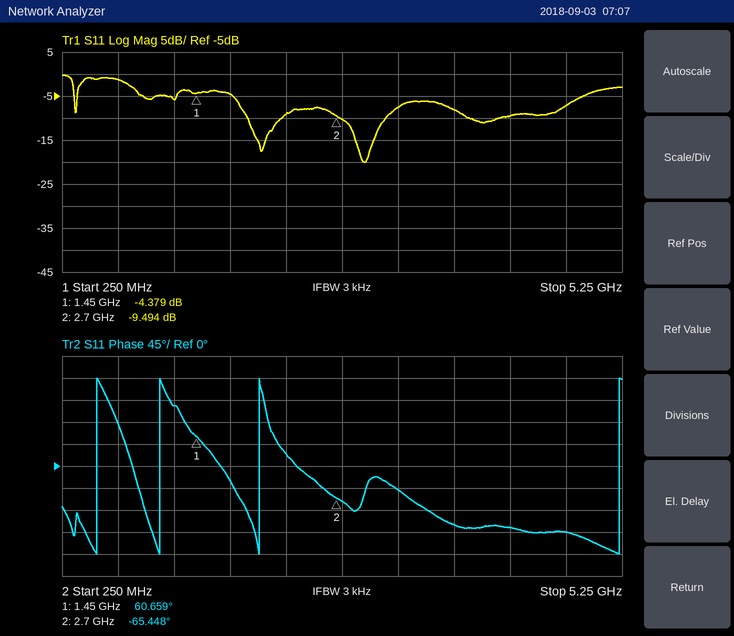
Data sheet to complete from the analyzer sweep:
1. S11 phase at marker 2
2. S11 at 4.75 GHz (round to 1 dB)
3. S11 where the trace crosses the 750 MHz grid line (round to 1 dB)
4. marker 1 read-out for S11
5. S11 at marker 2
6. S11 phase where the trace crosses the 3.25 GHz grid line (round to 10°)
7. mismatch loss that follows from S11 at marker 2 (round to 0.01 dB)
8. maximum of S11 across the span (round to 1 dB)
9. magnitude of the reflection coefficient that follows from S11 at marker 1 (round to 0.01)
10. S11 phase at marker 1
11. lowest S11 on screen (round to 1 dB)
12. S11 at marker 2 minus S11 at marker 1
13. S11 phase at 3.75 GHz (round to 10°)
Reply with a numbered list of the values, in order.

1. -65.448°
2. -7 dB
3. -1 dB
4. -4.379 dB
5. -9.494 dB
6. -50°
7. 0.52 dB
8. 0 dB
9. 0.60
10. 60.659°
11. -20 dB
12. -5.115 dB
13. -120°
